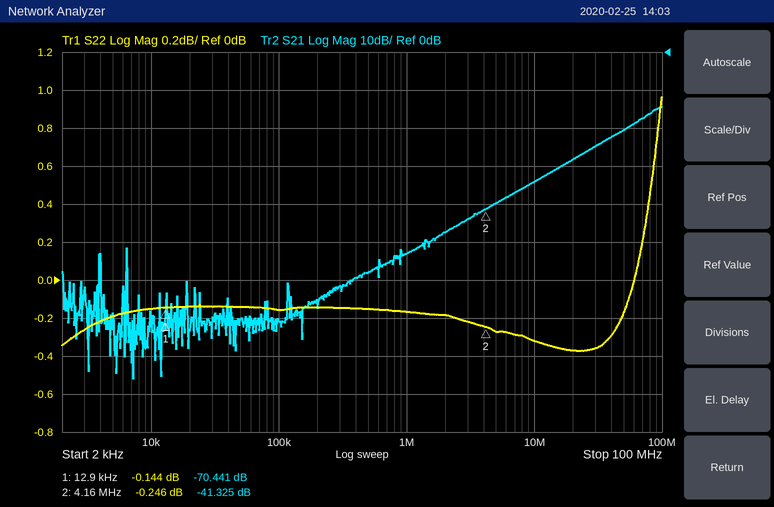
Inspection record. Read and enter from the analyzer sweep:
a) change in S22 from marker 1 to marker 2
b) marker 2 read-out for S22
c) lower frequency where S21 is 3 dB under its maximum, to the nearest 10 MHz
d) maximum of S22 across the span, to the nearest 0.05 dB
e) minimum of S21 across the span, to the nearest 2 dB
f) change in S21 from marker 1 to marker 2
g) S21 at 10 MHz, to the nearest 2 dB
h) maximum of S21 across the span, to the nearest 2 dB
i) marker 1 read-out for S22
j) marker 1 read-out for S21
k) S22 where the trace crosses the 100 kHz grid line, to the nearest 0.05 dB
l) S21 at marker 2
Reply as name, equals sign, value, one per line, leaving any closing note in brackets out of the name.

change in S22 from marker 1 to marker 2 = -0.102 dB
marker 2 read-out for S22 = -0.246 dB
lower frequency where S21 is 3 dB under its maximum, to the nearest 10 MHz = 70 MHz
maximum of S22 across the span, to the nearest 0.05 dB = 0.95 dB
minimum of S21 across the span, to the nearest 2 dB = -86 dB
change in S21 from marker 1 to marker 2 = 29.116 dB
S21 at 10 MHz, to the nearest 2 dB = -34 dB
maximum of S21 across the span, to the nearest 2 dB = -14 dB
marker 1 read-out for S22 = -0.144 dB
marker 1 read-out for S21 = -70.441 dB
S22 where the trace crosses the 100 kHz grid line, to the nearest 0.05 dB = -0.15 dB
S21 at marker 2 = -41.325 dB
